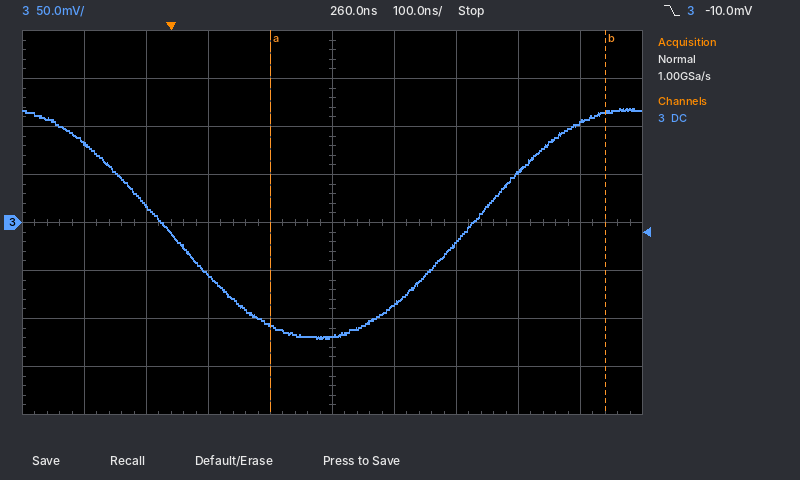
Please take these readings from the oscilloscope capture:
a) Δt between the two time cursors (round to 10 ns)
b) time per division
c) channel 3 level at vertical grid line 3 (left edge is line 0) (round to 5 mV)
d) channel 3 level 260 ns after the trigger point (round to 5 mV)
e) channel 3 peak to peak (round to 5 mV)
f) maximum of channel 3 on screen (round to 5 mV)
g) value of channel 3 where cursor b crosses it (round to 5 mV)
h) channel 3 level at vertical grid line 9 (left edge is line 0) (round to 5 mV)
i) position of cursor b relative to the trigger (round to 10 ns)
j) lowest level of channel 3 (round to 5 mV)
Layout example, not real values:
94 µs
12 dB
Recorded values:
540 ns
100 ns
-55 mV
-120 mV
240 mV
120 mV
115 mV
105 mV
+700 ns
-120 mV
